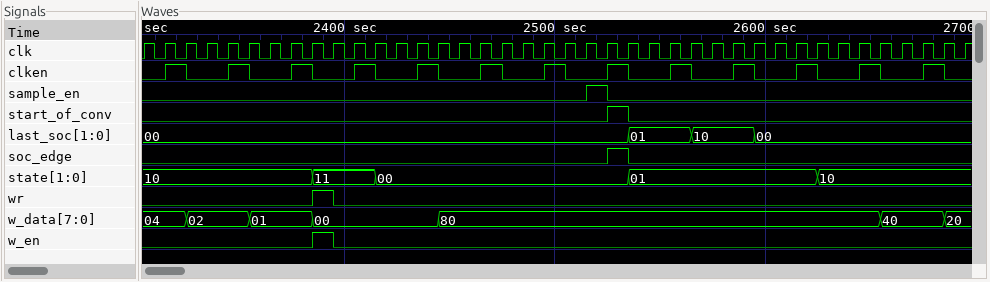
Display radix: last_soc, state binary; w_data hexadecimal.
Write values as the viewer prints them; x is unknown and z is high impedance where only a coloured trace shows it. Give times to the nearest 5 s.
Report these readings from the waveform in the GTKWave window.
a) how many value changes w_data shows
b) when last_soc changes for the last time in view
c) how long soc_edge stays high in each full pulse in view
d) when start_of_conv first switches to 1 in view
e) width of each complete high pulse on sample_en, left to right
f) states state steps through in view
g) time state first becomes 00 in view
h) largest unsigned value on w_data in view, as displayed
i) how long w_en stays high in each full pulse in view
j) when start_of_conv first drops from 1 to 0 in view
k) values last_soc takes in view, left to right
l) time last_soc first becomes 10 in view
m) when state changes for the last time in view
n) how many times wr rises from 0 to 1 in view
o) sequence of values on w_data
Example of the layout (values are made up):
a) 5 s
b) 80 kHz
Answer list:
a) 6
b) 2595 s
c) 10 s
d) 2525 s
e) 10 s
f) 10, 11, 00, 01, 10
g) 2415 s
h) 80
i) 10 s
j) 2535 s
k) 00, 01, 10, 00
l) 2565 s
m) 2625 s
n) 1
o) 04, 02, 01, 00, 80, 40, 20
